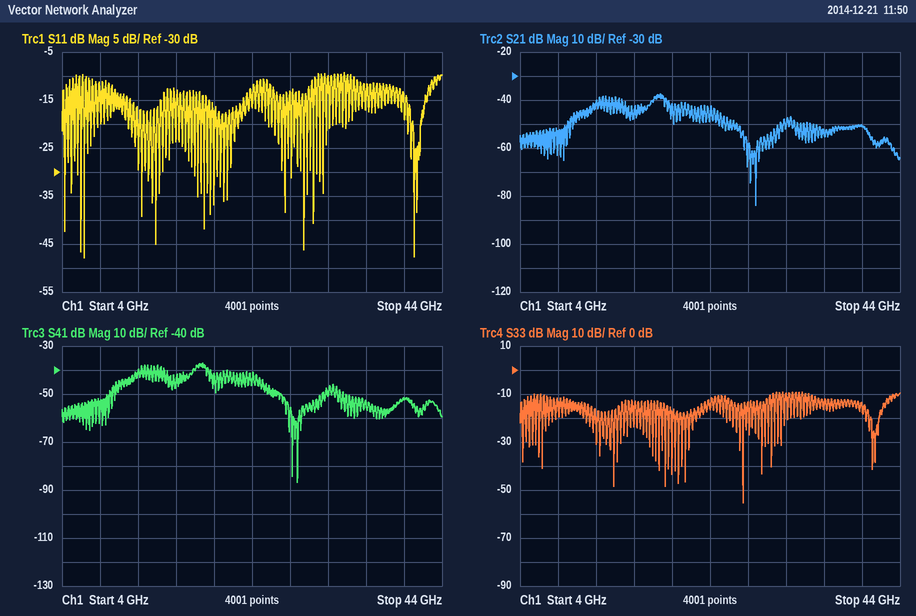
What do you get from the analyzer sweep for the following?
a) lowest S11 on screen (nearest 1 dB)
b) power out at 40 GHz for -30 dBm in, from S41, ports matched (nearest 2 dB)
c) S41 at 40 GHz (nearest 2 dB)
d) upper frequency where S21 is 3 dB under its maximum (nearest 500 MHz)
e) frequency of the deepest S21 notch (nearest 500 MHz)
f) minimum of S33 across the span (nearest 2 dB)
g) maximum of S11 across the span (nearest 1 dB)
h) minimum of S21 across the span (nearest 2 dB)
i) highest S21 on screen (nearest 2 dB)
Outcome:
-48 dB
-82 dBm
-52 dB
19.0 GHz
29.0 GHz
-56 dB
-9 dB
-84 dB
-38 dB
